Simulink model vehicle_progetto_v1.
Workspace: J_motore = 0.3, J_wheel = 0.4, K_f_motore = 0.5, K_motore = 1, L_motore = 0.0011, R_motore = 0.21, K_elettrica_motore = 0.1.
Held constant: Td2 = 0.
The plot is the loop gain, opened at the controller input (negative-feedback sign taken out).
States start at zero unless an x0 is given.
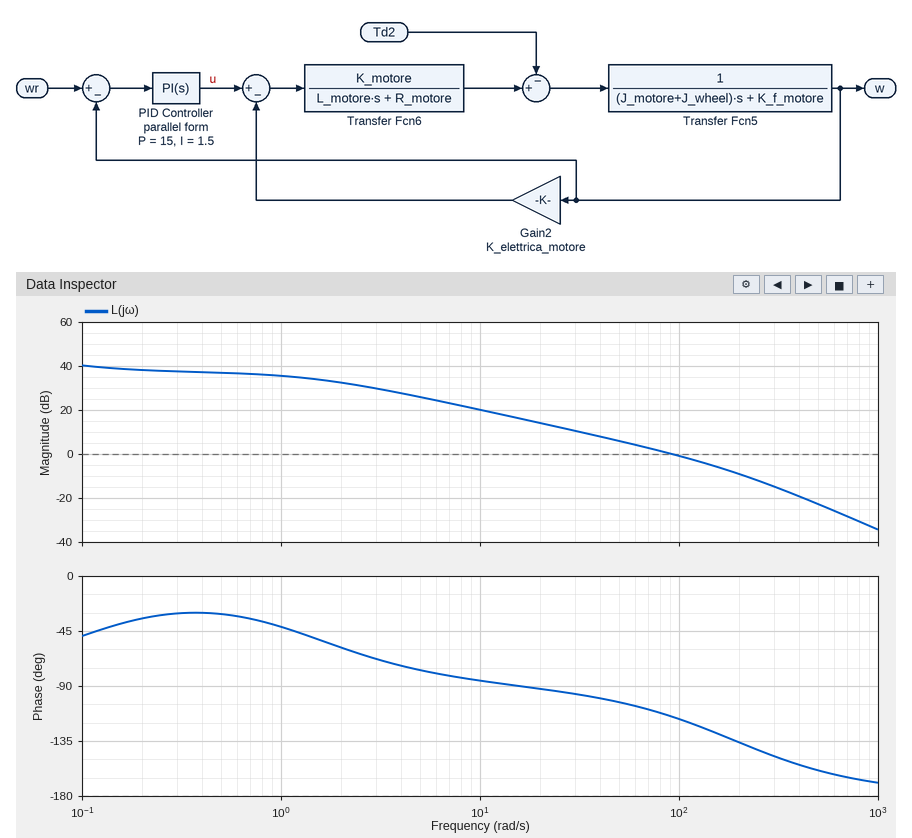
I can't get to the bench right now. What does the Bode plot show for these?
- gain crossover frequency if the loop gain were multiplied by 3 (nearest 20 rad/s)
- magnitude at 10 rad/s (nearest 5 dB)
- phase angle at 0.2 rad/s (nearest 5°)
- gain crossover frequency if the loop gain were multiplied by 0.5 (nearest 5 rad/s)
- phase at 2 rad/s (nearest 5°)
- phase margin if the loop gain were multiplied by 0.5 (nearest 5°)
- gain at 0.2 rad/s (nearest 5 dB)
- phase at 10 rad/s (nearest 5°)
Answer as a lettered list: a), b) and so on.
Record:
a) 200 rad/s
b) 20 dB
c) -35°
d) 50 rad/s
e) -60°
f) 75°
g) 40 dB
h) -85°
